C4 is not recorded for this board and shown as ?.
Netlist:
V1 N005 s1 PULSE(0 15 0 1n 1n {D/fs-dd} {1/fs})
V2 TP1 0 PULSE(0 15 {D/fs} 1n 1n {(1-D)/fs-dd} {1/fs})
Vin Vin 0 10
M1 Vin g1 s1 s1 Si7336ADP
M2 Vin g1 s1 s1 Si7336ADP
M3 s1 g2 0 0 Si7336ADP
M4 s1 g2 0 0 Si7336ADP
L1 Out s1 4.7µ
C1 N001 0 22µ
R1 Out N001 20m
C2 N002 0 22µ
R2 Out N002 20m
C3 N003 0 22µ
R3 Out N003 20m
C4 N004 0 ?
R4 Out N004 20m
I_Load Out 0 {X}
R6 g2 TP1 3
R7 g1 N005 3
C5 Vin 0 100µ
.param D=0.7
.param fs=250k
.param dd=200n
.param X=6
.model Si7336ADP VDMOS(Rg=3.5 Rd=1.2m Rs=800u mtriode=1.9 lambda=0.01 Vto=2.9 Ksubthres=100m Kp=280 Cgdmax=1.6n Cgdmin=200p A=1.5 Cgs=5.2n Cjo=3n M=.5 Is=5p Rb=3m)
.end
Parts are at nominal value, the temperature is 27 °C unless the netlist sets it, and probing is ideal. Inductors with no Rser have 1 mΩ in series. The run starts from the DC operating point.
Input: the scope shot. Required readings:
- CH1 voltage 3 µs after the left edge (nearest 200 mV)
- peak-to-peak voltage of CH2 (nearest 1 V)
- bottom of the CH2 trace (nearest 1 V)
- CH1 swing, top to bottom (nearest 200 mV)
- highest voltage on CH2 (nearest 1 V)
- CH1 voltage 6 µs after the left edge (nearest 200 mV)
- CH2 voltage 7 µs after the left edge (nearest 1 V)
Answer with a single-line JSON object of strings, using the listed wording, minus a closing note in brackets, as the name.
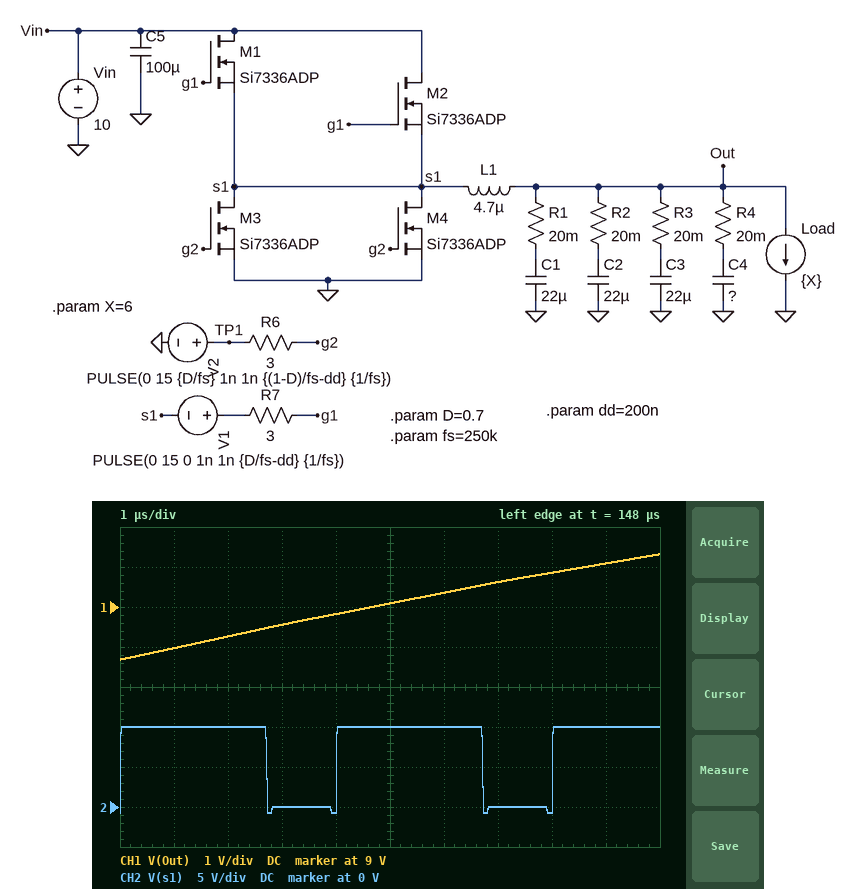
{"CH1 voltage 3 µs after the left edge": "8.6 V", "peak-to-peak voltage of CH2": "11 V", "bottom of the CH2 trace": "-1 V", "CH1 swing, top to bottom": "2.6 V", "highest voltage on CH2": "10 V", "CH1 voltage 6 µs after the left edge": "9.4 V", "CH2 voltage 7 µs after the left edge": "0 V"}
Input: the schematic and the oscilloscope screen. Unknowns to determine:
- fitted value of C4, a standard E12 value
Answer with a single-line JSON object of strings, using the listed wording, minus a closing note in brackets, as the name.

{"fitted value of C4, a standard E12 value": "6.8 µF"}
